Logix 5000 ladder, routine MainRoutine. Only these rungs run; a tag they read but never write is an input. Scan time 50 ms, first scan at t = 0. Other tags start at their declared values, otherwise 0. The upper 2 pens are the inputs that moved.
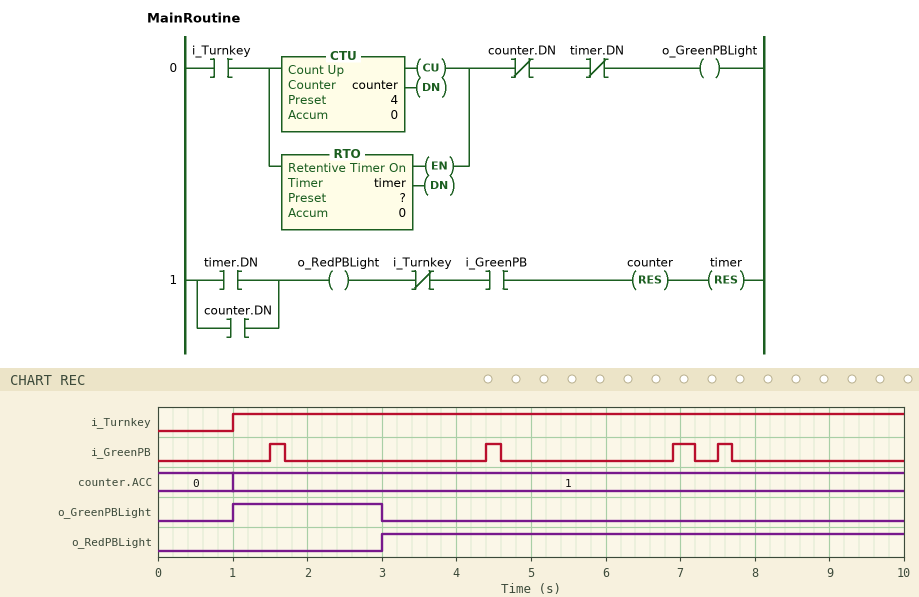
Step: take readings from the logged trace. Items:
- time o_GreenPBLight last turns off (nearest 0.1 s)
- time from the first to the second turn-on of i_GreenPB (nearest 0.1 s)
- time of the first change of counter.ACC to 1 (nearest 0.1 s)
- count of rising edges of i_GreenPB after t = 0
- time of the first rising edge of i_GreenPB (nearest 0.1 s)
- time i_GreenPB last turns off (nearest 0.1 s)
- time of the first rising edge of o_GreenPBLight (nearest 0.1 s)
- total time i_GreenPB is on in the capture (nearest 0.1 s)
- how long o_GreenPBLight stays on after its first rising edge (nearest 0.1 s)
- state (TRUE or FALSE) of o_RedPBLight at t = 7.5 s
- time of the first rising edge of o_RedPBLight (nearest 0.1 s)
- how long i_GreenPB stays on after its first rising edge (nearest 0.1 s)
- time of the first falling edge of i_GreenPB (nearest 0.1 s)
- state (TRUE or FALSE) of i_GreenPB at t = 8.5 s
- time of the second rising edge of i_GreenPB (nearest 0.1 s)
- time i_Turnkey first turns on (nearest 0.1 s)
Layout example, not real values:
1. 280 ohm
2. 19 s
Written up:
1. 3.0 s
2. 2.9 s
3. 1.0 s
4. 4
5. 1.5 s
6. 7.7 s
7. 1.0 s
8. 0.9 s
9. 2.0 s
10. TRUE
11. 3.0 s
12. 0.2 s
13. 1.7 s
14. FALSE
15. 4.4 s
16. 1.0 s
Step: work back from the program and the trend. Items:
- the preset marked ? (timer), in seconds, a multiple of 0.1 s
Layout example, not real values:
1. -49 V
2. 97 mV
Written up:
1. 2.0 s
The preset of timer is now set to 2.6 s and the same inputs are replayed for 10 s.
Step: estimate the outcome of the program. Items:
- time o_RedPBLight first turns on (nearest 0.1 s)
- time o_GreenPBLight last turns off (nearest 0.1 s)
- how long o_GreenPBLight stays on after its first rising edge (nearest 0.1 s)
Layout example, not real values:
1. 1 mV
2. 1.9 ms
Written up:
1. 3.6 s
2. 3.6 s
3. 2.6 s
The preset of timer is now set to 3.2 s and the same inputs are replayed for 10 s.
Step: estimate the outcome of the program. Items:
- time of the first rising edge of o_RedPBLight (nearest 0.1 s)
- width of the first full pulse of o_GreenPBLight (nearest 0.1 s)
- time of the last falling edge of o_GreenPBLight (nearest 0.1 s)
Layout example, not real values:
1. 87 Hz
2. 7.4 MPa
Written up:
1. 4.2 s
2. 3.2 s
3. 4.2 s
